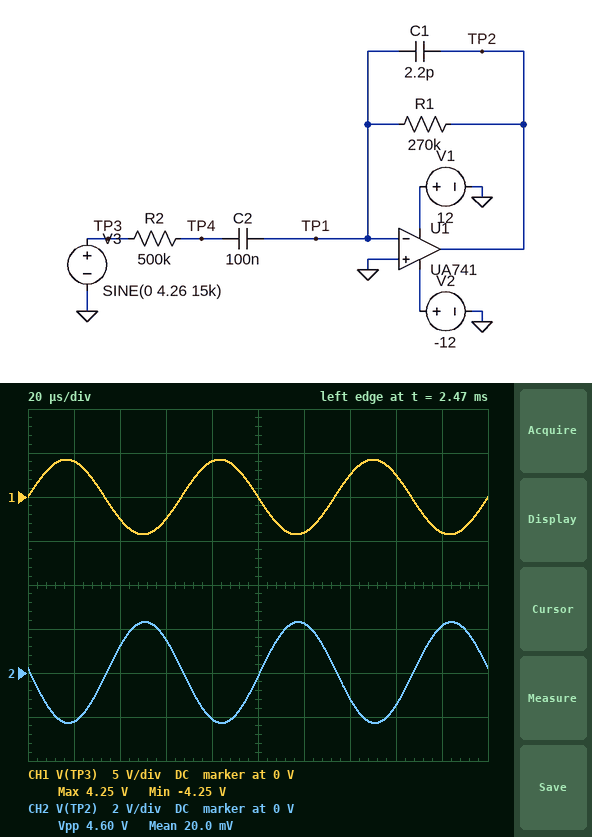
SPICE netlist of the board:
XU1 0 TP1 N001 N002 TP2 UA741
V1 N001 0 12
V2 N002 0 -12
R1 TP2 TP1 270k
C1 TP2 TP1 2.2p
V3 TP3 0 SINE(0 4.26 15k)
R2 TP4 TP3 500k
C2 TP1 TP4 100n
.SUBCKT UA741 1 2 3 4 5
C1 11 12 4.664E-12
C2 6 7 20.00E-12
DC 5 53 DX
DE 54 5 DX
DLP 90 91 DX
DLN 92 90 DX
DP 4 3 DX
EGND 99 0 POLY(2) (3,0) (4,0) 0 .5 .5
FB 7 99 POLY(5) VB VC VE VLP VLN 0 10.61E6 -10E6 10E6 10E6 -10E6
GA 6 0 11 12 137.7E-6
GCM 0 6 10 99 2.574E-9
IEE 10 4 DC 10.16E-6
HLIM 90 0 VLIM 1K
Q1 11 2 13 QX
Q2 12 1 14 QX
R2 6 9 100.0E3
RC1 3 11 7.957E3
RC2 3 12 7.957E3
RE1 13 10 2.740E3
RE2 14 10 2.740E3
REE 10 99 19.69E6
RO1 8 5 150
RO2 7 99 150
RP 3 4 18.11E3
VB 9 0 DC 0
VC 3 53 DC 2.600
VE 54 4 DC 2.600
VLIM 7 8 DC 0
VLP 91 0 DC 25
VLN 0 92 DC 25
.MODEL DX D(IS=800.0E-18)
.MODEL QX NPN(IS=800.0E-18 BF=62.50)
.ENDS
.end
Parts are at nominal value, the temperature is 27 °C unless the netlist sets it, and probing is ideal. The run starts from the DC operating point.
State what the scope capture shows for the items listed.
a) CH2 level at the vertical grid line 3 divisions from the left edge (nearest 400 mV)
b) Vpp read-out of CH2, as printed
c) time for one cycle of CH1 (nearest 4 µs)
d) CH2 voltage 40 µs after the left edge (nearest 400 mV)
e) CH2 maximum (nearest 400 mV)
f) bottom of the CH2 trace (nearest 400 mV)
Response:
1.6 V
4.60 V
68 µs
1.2 V
2.4 V
-2.4 V
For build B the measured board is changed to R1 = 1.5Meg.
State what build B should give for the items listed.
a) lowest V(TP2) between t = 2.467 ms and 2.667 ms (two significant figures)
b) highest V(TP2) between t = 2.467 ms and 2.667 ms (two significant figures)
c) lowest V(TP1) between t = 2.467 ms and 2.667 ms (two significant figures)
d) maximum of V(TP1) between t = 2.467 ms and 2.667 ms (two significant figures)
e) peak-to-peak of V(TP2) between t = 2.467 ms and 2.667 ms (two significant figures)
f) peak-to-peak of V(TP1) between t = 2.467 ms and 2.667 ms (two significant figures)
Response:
-8.4 V
8.6 V
-2.1 V
2.0 V
17 V
4.1 V
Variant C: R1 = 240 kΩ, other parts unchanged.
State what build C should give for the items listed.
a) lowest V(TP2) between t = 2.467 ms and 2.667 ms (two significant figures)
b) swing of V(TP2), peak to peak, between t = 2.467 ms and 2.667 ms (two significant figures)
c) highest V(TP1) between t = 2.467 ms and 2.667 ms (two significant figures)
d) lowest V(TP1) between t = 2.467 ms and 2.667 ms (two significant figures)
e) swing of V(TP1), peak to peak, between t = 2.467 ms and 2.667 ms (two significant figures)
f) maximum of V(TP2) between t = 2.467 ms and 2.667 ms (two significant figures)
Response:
-2.0 V
4.1 V
29 mV
-29 mV
58 mV
2.1 V
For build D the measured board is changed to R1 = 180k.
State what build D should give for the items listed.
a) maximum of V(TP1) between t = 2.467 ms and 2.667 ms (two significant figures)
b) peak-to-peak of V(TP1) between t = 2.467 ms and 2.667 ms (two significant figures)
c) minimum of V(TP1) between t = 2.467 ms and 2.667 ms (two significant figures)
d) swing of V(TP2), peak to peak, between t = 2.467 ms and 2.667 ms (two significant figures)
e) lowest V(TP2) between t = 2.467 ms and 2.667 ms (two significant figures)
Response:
21 mV
43 mV
-21 mV
3.1 V
-1.5 V
